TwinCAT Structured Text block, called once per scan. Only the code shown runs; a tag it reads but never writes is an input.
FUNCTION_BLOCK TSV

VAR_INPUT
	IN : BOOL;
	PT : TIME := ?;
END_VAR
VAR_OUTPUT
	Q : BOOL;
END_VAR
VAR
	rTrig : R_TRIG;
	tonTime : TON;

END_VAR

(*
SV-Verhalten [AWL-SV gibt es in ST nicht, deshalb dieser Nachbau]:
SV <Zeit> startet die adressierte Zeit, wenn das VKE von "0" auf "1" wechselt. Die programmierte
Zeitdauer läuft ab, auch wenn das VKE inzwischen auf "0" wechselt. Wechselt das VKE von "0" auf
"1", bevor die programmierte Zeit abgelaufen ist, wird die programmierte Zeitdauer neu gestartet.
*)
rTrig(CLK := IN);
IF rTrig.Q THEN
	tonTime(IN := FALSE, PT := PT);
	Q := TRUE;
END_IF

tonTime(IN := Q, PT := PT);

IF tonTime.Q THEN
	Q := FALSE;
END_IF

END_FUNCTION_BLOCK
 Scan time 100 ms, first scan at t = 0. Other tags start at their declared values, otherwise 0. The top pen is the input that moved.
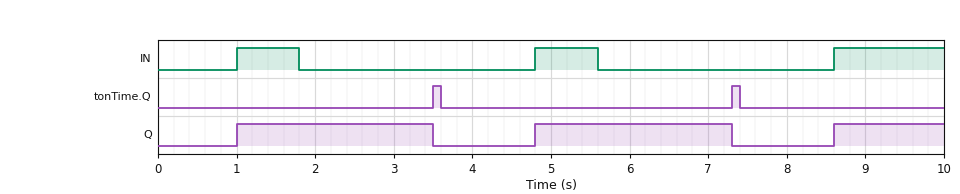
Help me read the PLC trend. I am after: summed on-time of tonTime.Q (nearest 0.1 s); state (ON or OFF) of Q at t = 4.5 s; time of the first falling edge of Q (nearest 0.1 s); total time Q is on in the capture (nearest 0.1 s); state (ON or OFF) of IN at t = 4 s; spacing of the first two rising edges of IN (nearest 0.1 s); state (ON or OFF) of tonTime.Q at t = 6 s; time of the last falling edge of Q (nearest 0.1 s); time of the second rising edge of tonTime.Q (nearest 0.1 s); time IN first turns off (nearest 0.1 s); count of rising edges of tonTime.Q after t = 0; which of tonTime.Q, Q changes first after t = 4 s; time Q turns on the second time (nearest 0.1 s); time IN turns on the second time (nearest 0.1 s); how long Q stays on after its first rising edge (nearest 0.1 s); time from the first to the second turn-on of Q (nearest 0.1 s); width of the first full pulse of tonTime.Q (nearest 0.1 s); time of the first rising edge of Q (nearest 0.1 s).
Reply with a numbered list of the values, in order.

1. 0.2 s
2. OFF
3. 3.5 s
4. 6.4 s
5. OFF
6. 3.8 s
7. OFF
8. 7.3 s
9. 7.3 s
10. 1.8 s
11. 2
12. Q
13. 4.8 s
14. 4.8 s
15. 2.5 s
16. 3.8 s
17. 0.1 s
18. 1.0 s
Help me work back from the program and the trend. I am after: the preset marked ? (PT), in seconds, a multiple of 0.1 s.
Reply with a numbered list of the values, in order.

1. 2.5 s
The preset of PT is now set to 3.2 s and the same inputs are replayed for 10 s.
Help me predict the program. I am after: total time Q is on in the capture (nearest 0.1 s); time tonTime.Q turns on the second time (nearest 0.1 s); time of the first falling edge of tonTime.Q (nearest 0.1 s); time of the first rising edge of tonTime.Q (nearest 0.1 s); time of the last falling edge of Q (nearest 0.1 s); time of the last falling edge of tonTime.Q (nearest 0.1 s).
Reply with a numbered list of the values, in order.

1. 7.8 s
2. 8.0 s
3. 4.3 s
4. 4.2 s
5. 8.0 s
6. 8.1 s
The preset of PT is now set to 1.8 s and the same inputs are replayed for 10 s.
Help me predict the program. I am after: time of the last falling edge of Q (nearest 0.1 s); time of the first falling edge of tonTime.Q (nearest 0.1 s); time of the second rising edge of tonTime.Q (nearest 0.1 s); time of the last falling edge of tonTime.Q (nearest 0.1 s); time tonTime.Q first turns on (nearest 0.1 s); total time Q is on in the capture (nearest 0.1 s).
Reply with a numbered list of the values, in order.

1. 6.6 s
2. 2.9 s
3. 6.6 s
4. 6.7 s
5. 2.8 s
6. 5.0 s
